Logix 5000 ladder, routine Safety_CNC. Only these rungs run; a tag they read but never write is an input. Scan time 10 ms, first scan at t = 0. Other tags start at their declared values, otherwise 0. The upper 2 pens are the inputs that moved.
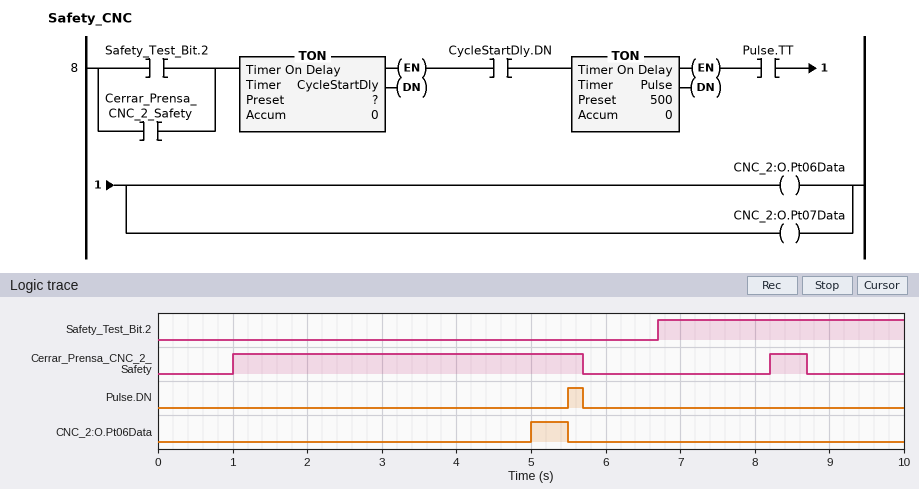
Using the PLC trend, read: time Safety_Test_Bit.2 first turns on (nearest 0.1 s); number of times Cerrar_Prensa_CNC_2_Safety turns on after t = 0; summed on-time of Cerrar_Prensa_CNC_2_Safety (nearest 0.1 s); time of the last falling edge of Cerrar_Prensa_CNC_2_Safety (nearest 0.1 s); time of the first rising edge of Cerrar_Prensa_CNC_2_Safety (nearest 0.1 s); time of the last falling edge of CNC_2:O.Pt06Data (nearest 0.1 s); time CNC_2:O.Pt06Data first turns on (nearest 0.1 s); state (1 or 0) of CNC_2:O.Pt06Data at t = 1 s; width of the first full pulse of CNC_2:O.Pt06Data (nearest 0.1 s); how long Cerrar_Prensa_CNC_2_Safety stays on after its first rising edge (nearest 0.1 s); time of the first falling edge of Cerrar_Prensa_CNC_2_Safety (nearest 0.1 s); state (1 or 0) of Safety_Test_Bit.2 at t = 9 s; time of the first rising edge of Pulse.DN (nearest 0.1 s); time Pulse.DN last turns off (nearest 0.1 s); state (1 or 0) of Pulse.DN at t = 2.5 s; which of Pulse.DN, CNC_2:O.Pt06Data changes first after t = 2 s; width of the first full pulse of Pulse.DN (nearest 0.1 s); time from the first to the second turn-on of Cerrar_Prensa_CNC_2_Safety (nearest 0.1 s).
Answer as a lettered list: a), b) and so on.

a) 6.7 s
b) 2
c) 5.2 s
d) 8.7 s
e) 1.0 s
f) 5.5 s
g) 5.0 s
h) 0
i) 0.5 s
j) 4.7 s
k) 5.7 s
l) 1
m) 5.5 s
n) 5.7 s
o) 0
p) CNC_2:O.Pt06Data
q) 0.2 s
r) 7.2 s
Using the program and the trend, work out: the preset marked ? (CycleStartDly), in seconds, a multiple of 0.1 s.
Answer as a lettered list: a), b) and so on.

a) 4.0 s
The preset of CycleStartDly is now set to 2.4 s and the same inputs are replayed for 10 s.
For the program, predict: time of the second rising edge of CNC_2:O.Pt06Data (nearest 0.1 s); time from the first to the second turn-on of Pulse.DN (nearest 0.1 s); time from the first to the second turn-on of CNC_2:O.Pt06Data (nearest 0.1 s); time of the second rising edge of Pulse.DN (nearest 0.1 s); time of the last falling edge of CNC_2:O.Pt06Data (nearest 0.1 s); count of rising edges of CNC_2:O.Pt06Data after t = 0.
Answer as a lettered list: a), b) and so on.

a) 9.1 s
b) 5.7 s
c) 5.7 s
d) 9.6 s
e) 9.6 s
f) 2
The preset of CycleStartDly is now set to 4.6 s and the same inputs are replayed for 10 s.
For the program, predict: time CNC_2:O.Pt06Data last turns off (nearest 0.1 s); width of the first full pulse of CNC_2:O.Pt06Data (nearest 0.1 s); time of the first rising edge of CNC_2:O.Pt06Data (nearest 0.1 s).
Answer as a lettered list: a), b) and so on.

a) 5.7 s
b) 0.1 s
c) 5.6 s
